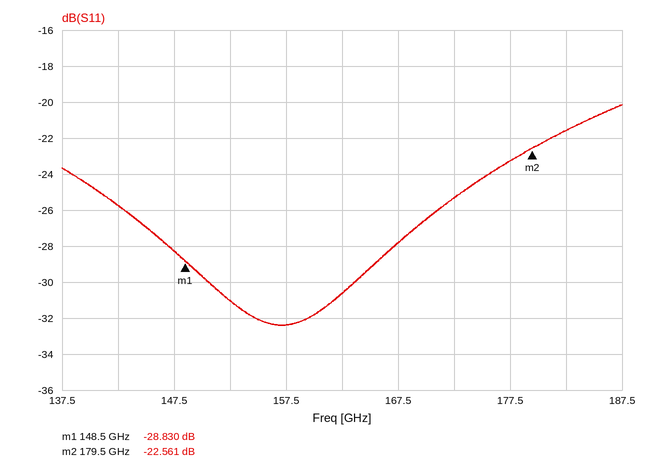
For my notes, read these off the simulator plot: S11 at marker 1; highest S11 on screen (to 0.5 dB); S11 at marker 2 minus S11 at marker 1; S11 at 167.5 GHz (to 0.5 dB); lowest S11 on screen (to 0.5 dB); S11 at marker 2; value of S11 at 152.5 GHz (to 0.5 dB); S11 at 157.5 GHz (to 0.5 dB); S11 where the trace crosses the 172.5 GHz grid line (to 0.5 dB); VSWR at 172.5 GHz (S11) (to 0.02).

-28.830 dB
-20.0 dB
6.269 dB
-28.0 dB
-32.5 dB
-22.561 dB
-31.0 dB
-32.5 dB
-25.5 dB
1.12
